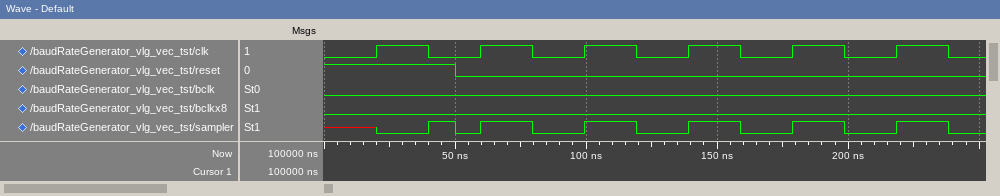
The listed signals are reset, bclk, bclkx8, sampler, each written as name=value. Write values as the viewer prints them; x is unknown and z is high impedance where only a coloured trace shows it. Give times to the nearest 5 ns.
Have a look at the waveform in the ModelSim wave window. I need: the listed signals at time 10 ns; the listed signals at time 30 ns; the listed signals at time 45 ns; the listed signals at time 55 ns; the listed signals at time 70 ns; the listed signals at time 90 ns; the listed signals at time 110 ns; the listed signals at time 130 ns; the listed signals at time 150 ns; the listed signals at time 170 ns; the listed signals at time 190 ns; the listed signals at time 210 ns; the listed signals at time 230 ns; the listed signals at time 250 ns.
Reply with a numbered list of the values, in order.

1. reset=1, bclk=0, bclkx8=0, sampler=x
2. reset=1, bclk=0, bclkx8=0, sampler=0
3. reset=1, bclk=0, bclkx8=0, sampler=1
4. reset=0, bclk=0, bclkx8=0, sampler=0
5. reset=0, bclk=0, bclkx8=0, sampler=1
6. reset=0, bclk=0, bclkx8=0, sampler=0
7. reset=0, bclk=0, bclkx8=0, sampler=1
8. reset=0, bclk=0, bclkx8=0, sampler=0
9. reset=0, bclk=0, bclkx8=0, sampler=1
10. reset=0, bclk=0, bclkx8=0, sampler=0
11. reset=0, bclk=0, bclkx8=0, sampler=1
12. reset=0, bclk=0, bclkx8=0, sampler=0
13. reset=0, bclk=0, bclkx8=0, sampler=1
14. reset=0, bclk=0, bclkx8=0, sampler=0
